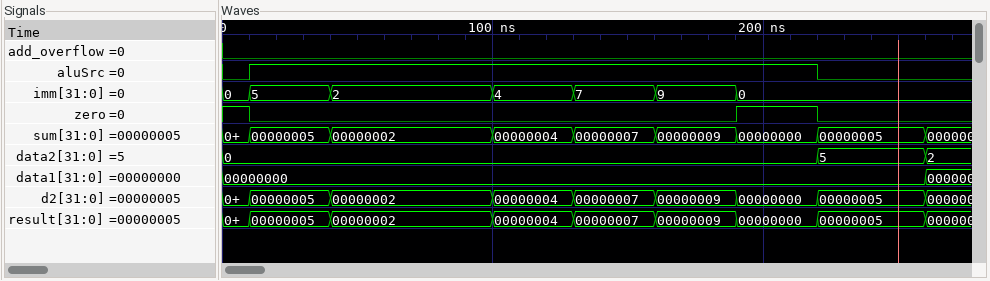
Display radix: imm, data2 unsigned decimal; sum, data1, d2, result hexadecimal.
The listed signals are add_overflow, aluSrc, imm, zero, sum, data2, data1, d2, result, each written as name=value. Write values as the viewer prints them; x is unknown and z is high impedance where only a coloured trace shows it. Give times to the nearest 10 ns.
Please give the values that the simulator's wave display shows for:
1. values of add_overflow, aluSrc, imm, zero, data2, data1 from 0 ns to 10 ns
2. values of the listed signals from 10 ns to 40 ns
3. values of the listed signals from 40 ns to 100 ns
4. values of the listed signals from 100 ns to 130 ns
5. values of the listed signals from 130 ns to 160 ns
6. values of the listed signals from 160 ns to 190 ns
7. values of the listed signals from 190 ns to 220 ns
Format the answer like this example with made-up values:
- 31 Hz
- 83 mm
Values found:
- add_overflow=0, aluSrc=0, imm=0, zero=1, data2=0, data1=00000000
- add_overflow=0, aluSrc=1, imm=5, zero=0, sum=00000005, data2=0, data1=00000000, d2=00000005, result=00000005
- add_overflow=0, aluSrc=1, imm=2, zero=0, sum=00000002, data2=0, data1=00000000, d2=00000002, result=00000002
- add_overflow=0, aluSrc=1, imm=4, zero=0, sum=00000004, data2=0, data1=00000000, d2=00000004, result=00000004
- add_overflow=0, aluSrc=1, imm=7, zero=0, sum=00000007, data2=0, data1=00000000, d2=00000007, result=00000007
- add_overflow=0, aluSrc=1, imm=9, zero=0, sum=00000009, data2=0, data1=00000000, d2=00000009, result=00000009
- add_overflow=0, aluSrc=1, imm=0, zero=1, sum=00000000, data2=0, data1=00000000, d2=00000000, result=00000000
